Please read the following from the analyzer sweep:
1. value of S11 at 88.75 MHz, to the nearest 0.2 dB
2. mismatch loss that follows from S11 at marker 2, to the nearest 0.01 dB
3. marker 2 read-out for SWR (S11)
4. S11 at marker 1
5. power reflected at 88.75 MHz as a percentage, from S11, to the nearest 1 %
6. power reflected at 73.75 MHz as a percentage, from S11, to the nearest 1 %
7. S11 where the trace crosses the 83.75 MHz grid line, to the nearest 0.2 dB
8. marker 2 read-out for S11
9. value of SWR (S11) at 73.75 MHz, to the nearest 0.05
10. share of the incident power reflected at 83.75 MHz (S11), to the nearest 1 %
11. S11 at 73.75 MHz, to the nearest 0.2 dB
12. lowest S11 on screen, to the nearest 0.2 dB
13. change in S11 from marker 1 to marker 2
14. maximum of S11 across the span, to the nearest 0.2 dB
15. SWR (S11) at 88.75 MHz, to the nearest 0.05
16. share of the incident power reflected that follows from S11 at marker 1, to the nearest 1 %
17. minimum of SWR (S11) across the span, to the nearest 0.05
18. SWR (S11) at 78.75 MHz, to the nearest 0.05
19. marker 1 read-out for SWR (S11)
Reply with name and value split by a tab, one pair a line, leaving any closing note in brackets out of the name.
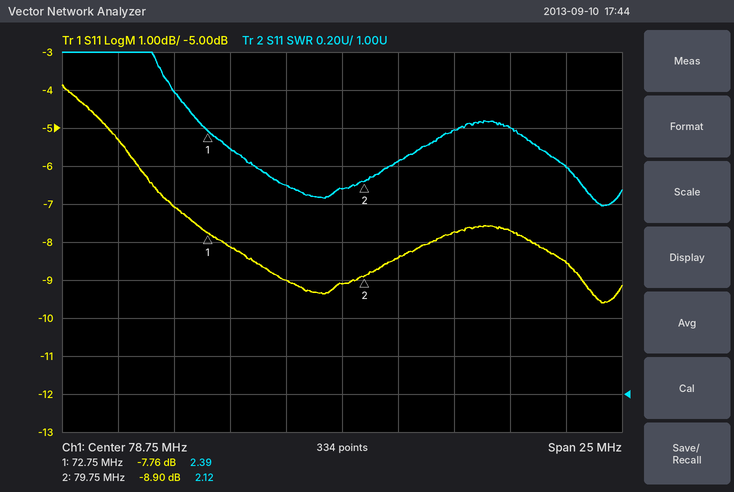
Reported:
value of S11 at 88.75 MHz, to the nearest 0.2 dB	-8.6 dB
mismatch loss that follows from S11 at marker 2, to the nearest 0.01 dB	0.60 dB
marker 2 read-out for SWR	2.12
S11 at marker 1	-7.76 dB
power reflected at 88.75 MHz as a percentage, from S11, to the nearest 1 %	14 %
power reflected at 73.75 MHz as a percentage, from S11, to the nearest 1 %	15 %
S11 where the trace crosses the 83.75 MHz grid line, to the nearest 0.2 dB	-7.8 dB
marker 2 read-out for S11	-8.90 dB
value of SWR (S11) at 73.75 MHz, to the nearest 0.05	2.30
share of the incident power reflected at 83.75 MHz (S11), to the nearest 1 %	17 %
S11 at 73.75 MHz, to the nearest 0.2 dB	-8.2 dB
lowest S11 on screen, to the nearest 0.2 dB	-9.6 dB
change in S11 from marker 1 to marker 2	-1.14 dB
maximum of S11 across the span, to the nearest 0.2 dB	-3.8 dB
SWR (S11) at 88.75 MHz, to the nearest 0.05	2.20
share of the incident power reflected that follows from S11 at marker 1, to the nearest 1 %	17 %
minimum of SWR (S11) across the span, to the nearest 0.05	2.00
SWR (S11) at 78.75 MHz, to the nearest 0.05	2.10
marker 1 read-out for SWR	2.39
